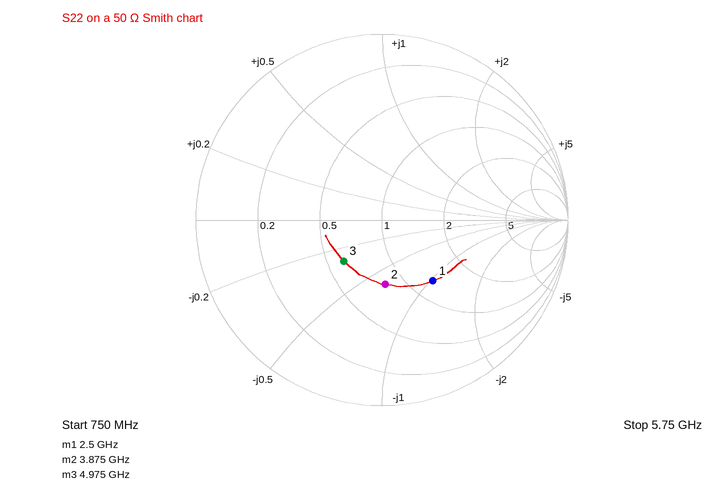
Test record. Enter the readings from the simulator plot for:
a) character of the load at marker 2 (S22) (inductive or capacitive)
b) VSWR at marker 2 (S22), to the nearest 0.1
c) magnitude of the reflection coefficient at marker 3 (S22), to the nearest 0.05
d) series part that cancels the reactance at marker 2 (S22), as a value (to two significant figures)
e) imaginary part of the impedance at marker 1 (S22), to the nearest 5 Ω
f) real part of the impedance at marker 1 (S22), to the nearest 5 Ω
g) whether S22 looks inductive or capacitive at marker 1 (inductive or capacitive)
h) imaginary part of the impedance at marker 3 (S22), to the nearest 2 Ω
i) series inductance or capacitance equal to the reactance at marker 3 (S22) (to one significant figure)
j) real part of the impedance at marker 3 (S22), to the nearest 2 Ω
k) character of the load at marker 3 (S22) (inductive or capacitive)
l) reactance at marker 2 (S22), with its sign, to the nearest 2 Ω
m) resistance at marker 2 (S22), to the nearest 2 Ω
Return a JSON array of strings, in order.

["capacitive", "2.1", "0.30", "1.3 nH", "-50 Ω", "65 Ω", "capacitive", "-14 Ω", "2 pF", "30 Ω", "capacitive", "-32 Ω", "40 Ω"]
